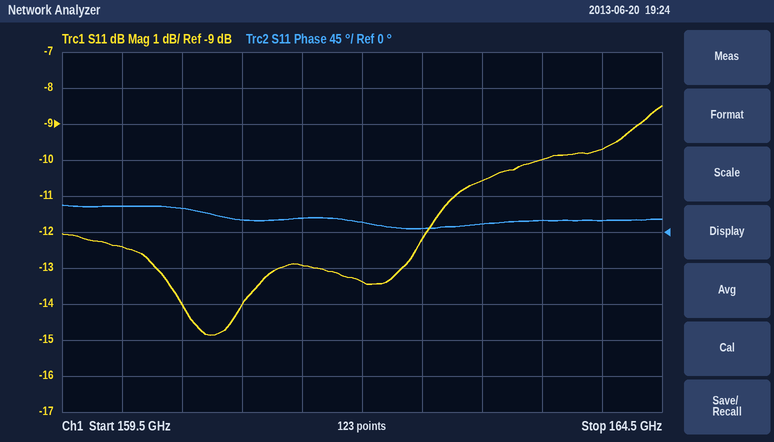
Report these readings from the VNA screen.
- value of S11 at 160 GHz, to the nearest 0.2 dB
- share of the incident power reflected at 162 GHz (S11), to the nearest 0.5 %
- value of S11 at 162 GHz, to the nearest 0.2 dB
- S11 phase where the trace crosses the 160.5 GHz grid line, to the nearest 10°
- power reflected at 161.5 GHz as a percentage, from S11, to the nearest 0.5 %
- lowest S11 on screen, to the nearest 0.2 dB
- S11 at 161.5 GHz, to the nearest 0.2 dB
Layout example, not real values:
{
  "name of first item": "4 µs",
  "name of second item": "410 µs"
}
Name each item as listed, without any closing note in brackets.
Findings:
{
  "value of S11 at 160 GHz, to the nearest 0.2 dB": "-12.4 dB",
  "share of the incident power reflected at 162 GHz (S11), to the nearest 0.5 %": "4.5 %",
  "value of S11 at 162 GHz, to the nearest 0.2 dB": "-13.4 dB",
  "S11 phase where the trace crosses the 160.5 GHz grid line, to the nearest 10°": "30°",
  "power reflected at 161.5 GHz as a percentage, from S11, to the nearest 0.5 %": "5.0 %",
  "lowest S11 on screen, to the nearest 0.2 dB": "-14.8 dB",
  "S11 at 161.5 GHz, to the nearest 0.2 dB": "-13.0 dB"
}
